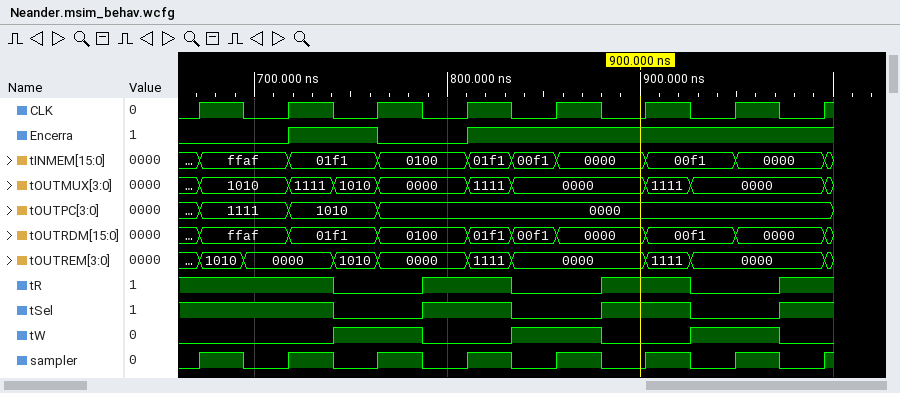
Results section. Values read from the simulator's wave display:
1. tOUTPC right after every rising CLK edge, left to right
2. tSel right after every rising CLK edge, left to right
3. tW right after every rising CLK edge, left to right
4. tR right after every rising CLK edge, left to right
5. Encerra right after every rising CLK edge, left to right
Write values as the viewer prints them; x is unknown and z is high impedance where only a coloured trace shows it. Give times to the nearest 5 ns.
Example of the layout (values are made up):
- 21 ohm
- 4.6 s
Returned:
- 1111, 1010, 0000, 0000, 0000, 0000, 0000, 0000
- 1 1 0 1 0 1 0 1
- 0 0 1 0 1 0 1 0
- 1 1 0 1 0 1 0 1
- 0 1 0 1 1 1 1 1
